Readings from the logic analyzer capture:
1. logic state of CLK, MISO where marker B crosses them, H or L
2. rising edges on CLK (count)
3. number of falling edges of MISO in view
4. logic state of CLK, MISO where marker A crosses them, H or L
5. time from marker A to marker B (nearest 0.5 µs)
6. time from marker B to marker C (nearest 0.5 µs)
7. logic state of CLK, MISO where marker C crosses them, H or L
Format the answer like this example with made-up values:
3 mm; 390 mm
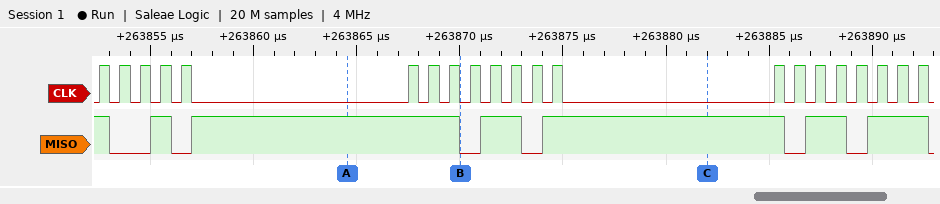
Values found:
CLK=L, MISO=L; 21; 7; CLK=L, MISO=H; 5.5 µs; 12 µs; CLK=L, MISO=H
